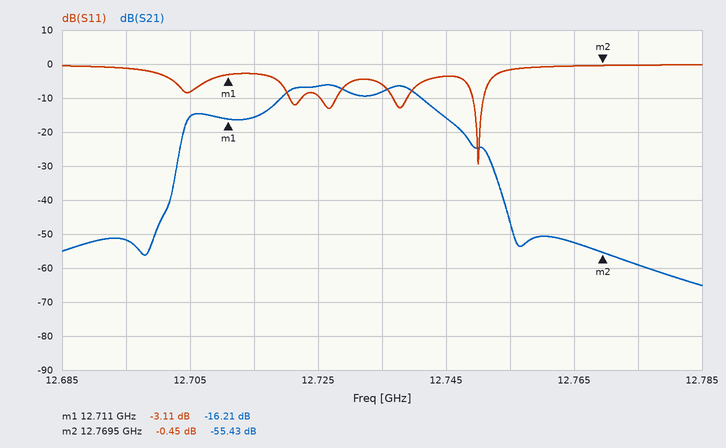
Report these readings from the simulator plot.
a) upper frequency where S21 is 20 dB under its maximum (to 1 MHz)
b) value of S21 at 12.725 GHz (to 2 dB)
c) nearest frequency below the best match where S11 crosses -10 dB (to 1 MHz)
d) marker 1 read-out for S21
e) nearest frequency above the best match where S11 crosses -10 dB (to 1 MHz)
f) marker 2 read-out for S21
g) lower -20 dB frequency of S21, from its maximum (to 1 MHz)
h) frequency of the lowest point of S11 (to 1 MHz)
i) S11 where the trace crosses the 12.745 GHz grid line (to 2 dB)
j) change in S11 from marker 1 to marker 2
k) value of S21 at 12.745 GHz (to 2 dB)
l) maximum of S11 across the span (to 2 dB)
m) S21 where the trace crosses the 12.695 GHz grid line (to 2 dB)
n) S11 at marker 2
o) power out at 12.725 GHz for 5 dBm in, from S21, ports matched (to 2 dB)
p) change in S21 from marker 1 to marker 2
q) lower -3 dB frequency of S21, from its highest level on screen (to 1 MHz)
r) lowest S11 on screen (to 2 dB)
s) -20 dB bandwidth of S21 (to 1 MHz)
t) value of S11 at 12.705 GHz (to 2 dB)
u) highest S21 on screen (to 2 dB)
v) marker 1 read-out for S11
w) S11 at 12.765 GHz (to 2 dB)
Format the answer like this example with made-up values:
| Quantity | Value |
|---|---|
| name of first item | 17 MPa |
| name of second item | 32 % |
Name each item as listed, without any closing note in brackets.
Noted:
| Quantity | Value |
|---|---|
| upper frequency where S21 is 20 dB under its maximum | 12.751 GHz |
| value of S21 at 12.725 GHz | -6 dB |
| nearest frequency below the best match where S11 crosses -10 dB | 12.749 GHz |
| marker 1 read-out for S21 | -16.21 dB |
| nearest frequency above the best match where S11 crosses -10 dB | 12.751 GHz |
| marker 2 read-out for S21 | -55.43 dB |
| lower -20 dB frequency of S21, from its maximum | 12.703 GHz |
| frequency of the lowest point of S11 | 12.750 GHz |
| S11 where the trace crosses the 12.745 GHz grid line | -4 dB |
| change in S11 from marker 1 to marker 2 | 2.66 dB |
| value of S21 at 12.745 GHz | -16 dB |
| maximum of S11 across the span | 0 dB |
| S21 where the trace crosses the 12.695 GHz grid line | -52 dB |
| S11 at marker 2 | -0.45 dB |
| power out at 12.725 GHz for 5 dBm in, from S21, ports matched | -2 dBm |
| change in S21 from marker 1 to marker 2 | -39.22 dB |
| lower -3 dB frequency of S21, from its highest level on screen | 12.720 GHz |
| lowest S11 on screen | -30 dB |
| -20 dB bandwidth of S21 | 48 MHz |
| value of S11 at 12.705 GHz | -8 dB |
| highest S21 on screen | -6 dB |
| marker 1 read-out for S11 | -3.11 dB |
| S11 at 12.765 GHz | 0 dB |
